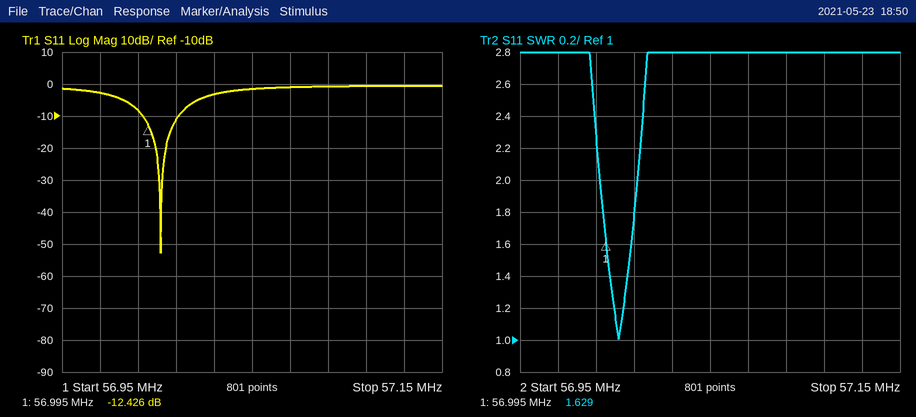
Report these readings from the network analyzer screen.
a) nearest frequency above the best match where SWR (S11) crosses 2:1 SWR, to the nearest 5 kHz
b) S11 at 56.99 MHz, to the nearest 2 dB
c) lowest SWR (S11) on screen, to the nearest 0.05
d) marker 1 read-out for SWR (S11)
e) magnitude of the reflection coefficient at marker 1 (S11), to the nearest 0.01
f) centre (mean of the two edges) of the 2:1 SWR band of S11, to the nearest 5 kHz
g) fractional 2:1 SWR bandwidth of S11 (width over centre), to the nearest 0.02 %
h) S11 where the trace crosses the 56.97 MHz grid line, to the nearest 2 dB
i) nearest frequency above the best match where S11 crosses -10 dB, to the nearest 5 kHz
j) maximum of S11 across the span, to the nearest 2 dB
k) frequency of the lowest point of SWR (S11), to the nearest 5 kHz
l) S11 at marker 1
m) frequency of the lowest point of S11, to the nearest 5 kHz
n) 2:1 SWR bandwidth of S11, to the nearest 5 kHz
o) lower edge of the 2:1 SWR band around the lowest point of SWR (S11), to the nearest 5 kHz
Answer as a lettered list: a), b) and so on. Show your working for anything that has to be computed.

a) 57.010 MHz
b) -8 dB
c) 1.00
d) 1.629
e) 10^(-12.426/20) ≈ 0.24
f) 57.000 MHz
g) 20 kHz / 57 MHz ≈ 0.04 %
h) -2 dB
i) 57.010 MHz
j) 0 dB
k) 57.000 MHz
l) -12.426 dB
m) 57.000 MHz
n) 57.010 MHz − 56.990 MHz = 20 kHz
o) 56.990 MHz
